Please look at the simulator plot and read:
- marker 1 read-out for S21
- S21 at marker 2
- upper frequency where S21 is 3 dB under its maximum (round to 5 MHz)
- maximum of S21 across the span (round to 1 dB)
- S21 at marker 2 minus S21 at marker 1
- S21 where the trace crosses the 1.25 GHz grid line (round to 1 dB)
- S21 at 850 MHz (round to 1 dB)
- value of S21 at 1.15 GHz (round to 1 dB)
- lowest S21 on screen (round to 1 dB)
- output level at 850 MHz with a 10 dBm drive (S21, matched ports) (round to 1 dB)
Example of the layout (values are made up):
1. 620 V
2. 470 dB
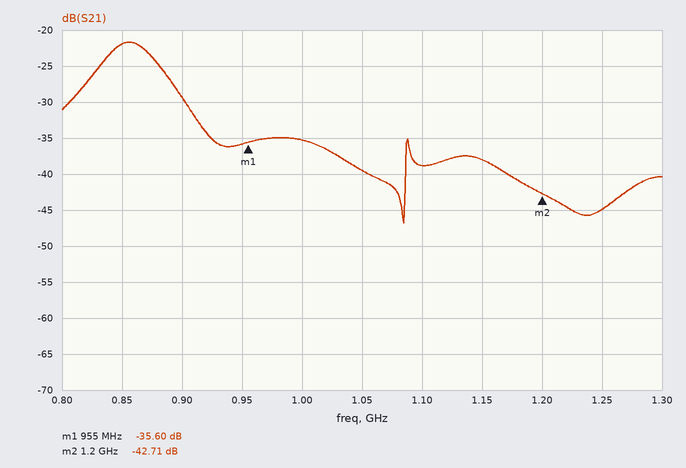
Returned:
1. -35.60 dB
2. -42.71 dB
3. 880 MHz
4. -22 dB
5. -7.11 dB
6. -45 dB
7. -22 dB
8. -38 dB
9. -47 dB
10. -12 dBm
